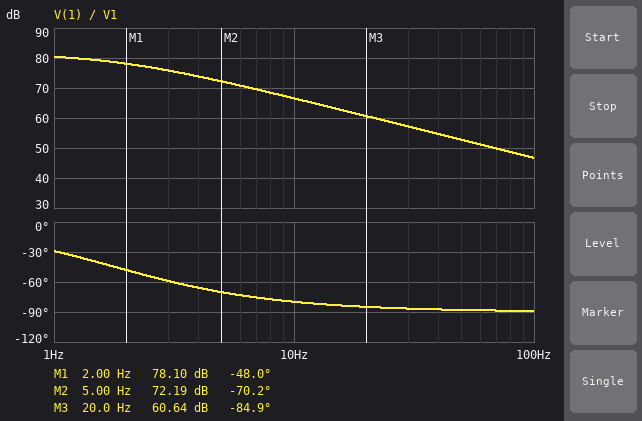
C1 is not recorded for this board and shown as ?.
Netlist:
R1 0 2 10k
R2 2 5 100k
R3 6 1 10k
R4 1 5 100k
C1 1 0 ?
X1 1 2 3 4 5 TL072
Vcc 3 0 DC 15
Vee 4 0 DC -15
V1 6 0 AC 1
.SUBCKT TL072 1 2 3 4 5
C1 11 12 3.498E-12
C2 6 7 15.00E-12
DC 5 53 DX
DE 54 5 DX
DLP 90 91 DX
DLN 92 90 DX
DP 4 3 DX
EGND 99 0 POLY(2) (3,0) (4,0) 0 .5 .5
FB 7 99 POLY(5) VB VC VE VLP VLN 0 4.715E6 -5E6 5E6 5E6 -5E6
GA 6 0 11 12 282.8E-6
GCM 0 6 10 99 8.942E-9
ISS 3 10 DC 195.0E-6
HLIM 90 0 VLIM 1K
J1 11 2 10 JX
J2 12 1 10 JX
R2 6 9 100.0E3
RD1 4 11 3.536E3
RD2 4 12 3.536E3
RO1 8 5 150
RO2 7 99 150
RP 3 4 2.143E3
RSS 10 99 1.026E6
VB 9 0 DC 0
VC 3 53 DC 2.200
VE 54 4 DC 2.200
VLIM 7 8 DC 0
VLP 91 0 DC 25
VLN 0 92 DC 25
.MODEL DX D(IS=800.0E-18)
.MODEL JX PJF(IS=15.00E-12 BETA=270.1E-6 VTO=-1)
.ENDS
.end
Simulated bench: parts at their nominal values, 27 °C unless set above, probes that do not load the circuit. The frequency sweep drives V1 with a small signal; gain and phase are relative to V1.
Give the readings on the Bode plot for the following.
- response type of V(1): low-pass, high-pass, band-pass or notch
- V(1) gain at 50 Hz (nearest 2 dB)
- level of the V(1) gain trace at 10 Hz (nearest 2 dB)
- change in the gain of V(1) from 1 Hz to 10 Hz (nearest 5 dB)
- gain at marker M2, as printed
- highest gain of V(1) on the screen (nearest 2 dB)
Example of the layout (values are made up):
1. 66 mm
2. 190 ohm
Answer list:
1. low-pass
2. 52 dB
3. 66 dB
4. -15 dB
5. 72.19 dB
6. 80 dB
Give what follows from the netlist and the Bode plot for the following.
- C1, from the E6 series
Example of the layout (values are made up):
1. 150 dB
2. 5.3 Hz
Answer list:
1. 680 pF
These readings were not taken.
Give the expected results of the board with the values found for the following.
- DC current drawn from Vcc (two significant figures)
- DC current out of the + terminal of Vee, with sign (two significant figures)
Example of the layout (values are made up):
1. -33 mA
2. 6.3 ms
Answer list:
1. 14 mA
2. -14 mA
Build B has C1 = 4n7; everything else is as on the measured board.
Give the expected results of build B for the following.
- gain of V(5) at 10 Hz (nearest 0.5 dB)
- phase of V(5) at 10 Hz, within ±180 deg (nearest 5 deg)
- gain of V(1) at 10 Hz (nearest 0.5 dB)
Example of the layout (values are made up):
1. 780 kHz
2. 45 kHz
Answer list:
1. 71.5 dB
2. -90 deg
3. 50.5 dB
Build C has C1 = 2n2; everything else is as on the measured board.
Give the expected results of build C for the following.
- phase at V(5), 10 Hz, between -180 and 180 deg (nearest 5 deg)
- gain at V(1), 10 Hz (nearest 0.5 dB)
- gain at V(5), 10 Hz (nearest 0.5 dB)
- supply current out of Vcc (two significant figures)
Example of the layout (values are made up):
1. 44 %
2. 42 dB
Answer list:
1. -85 deg
2. 57.0 dB
3. 78.0 dB
4. 14 mA
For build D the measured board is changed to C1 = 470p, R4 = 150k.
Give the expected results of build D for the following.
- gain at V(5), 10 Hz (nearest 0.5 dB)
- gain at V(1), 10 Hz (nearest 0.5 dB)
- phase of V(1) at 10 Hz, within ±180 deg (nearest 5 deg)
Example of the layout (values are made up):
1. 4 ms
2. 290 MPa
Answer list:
1. 30.5 dB
2. 9.5 dB
3. 0 deg
